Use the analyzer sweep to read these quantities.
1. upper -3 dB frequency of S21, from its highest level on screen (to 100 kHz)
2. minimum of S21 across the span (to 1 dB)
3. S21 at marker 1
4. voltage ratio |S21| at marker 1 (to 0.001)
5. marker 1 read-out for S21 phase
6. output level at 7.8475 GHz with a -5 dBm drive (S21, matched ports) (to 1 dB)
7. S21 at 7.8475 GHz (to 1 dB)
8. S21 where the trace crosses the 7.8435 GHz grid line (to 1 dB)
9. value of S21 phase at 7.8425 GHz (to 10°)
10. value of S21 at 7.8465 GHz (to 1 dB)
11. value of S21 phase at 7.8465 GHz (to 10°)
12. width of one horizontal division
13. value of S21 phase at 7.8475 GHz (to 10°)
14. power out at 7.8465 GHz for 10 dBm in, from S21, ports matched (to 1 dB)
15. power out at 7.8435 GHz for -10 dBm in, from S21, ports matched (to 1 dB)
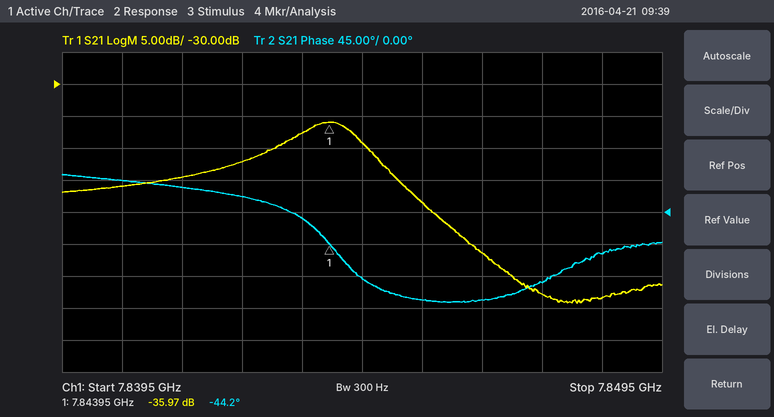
7.8445 GHz
-64 dB
-35.97 dB
0.016
-44.2°
-68 dBm
-63 dB
-38 dB
20°
-56 dB
-120°
1 MHz
-100°
-46 dBm
-48 dBm
